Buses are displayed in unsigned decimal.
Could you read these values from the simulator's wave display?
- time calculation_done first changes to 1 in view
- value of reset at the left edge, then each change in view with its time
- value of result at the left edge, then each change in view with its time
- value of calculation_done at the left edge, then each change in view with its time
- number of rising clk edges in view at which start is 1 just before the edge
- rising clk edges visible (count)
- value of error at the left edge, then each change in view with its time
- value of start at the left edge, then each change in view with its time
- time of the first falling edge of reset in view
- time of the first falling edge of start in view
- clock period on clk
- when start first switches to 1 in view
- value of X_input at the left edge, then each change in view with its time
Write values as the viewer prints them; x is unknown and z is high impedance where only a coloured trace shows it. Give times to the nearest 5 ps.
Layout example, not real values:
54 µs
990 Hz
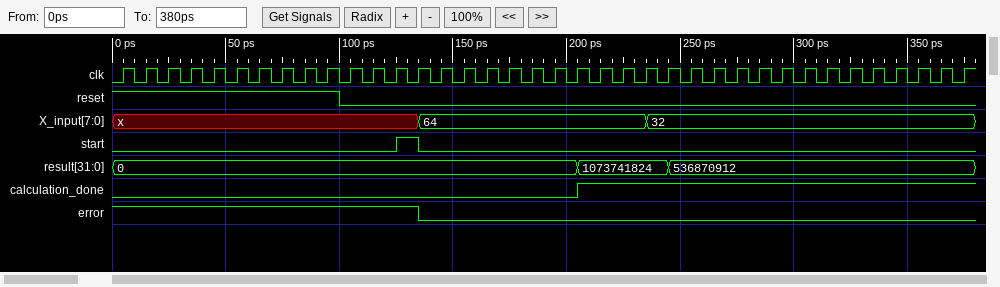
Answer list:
205 ps
1, 0 at 100 ps
0, 1073741824 at 205 ps, 536870912 at 245 ps
0, 1 at 205 ps
1
38
1, 0 at 135 ps
0, 1 at 125 ps, 0 at 135 ps
100 ps
135 ps
10 ps
125 ps
x, 64 at 135 ps, 32 at 235 ps
